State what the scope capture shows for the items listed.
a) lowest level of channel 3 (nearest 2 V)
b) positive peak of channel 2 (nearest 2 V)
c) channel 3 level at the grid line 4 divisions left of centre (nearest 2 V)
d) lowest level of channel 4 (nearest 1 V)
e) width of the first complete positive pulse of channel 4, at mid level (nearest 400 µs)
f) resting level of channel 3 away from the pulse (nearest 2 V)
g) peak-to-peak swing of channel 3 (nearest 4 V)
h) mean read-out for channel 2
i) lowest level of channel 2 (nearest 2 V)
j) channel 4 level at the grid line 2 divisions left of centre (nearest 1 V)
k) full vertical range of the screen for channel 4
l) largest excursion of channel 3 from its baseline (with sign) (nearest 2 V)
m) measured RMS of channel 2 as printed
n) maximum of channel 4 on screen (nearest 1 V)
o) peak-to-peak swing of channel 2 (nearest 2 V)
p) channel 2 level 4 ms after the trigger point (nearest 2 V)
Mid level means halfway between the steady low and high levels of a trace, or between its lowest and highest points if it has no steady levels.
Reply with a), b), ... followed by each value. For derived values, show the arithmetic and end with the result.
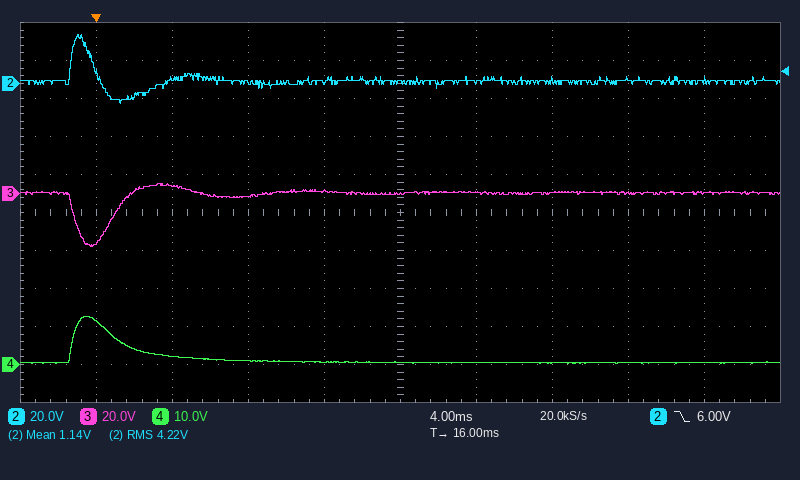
a) -28 V
b) 26 V
c) -26 V
d) 0 V
e) 2.4 ms
f) 0 V
g) 32 V
h) 1.14 V
i) -10 V
j) 1 V
k) 100 V
l) -28 V − (0 V) = -28 V
m) 4.22 V
n) 13 V
o) 26 V − (-10 V) = 36 V
p) 2 V
